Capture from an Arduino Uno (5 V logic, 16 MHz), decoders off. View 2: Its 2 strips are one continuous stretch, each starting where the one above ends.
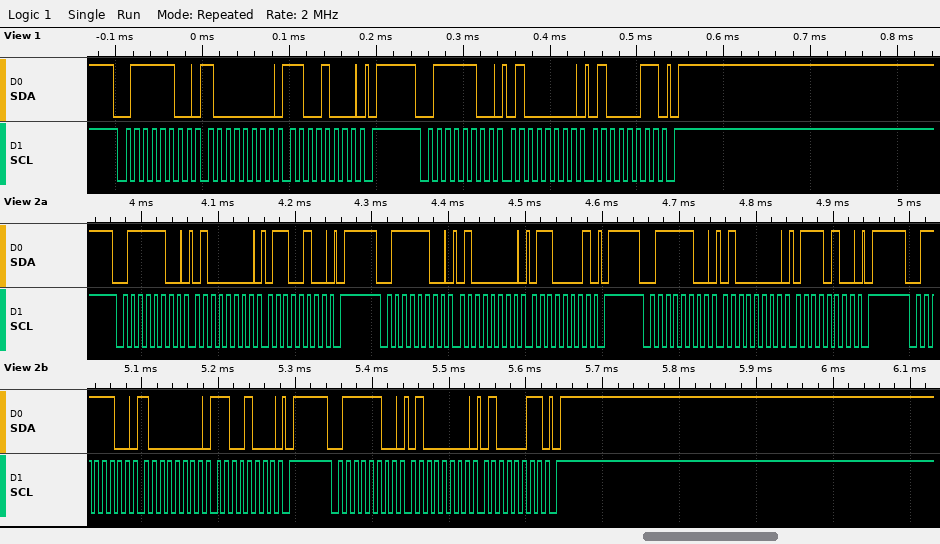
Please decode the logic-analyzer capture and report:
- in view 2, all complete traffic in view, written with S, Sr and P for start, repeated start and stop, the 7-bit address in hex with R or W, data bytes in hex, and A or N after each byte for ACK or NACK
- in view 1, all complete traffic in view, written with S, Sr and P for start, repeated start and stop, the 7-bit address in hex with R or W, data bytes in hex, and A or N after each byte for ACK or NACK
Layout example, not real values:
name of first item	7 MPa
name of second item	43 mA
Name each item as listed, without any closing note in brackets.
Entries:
in view 2, all complete traffic in view, written with S, Sr and P for start, repeated start and stop, the 7-bit address in hex with R or W, data bytes in hex, and A or N after each byte for ACK or NACK	S 3EW A 40 A 64 A P S 3EW A 40 A 61 A P S 3EW A 40 A 74 A P S 3EW A 80 A C8 A P S 3EW A 40 A 43 A P
in view 1, all complete traffic in view, written with S, Sr and P for start, repeated start and stop, the 7-bit address in hex with R or W, data bytes in hex, and A or N after each byte for ACK or NACK	S 3EW A 80 A C8 A P S 3EW A 40 A 43 A P
